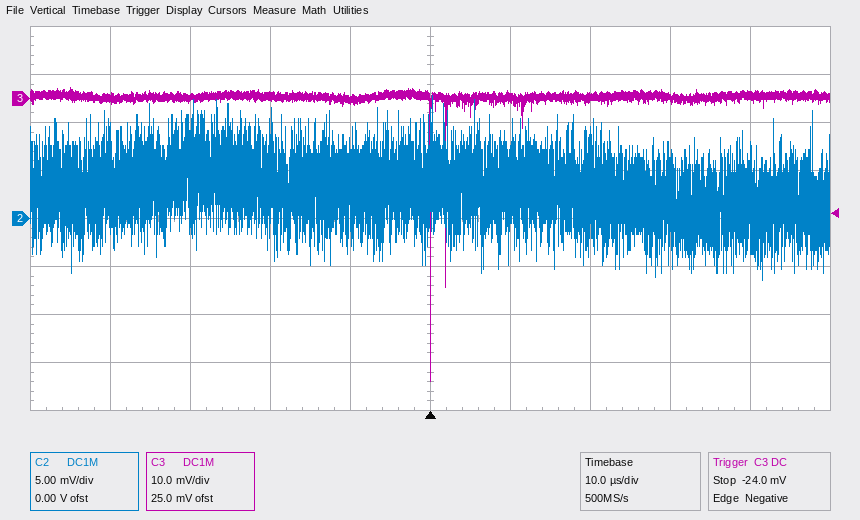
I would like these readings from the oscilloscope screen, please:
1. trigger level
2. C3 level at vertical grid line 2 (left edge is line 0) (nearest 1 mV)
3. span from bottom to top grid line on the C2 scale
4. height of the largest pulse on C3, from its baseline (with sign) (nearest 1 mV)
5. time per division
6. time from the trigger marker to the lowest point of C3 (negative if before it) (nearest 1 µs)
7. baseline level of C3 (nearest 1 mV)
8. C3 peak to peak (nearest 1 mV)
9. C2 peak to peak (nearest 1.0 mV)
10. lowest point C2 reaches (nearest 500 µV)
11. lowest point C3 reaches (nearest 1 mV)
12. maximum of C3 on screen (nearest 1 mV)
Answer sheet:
-24.0 mV
0 mV
40 mV
-59 mV
10 µs
0 µs
0 mV
61 mV
19.0 mV
-6.5 mV
-59 mV
2 mV
